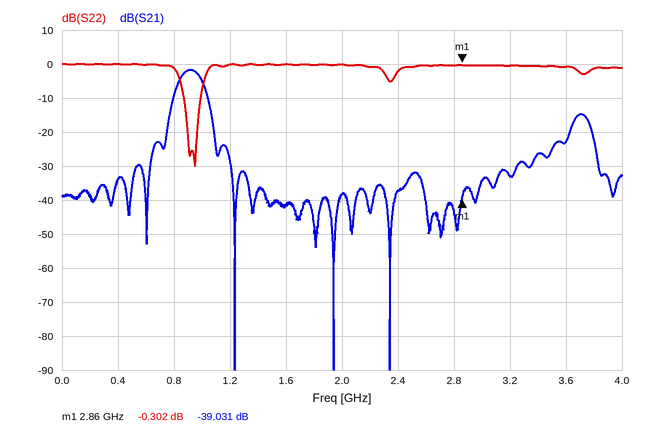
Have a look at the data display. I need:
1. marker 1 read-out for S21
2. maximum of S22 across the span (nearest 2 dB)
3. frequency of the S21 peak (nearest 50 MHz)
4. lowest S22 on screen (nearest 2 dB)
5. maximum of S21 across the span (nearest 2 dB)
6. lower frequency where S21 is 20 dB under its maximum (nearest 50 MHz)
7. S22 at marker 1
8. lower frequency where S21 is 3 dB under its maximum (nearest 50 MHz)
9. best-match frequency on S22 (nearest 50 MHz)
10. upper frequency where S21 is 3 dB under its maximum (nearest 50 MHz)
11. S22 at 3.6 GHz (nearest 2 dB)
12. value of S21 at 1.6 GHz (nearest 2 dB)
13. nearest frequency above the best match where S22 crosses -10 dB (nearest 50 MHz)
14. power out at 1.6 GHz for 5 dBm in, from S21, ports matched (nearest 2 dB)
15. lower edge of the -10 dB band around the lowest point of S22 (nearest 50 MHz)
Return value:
-39.031 dB
0 dB
900 MHz
-30 dB
-2 dB
750 MHz
-0.302 dB
850 MHz
950 MHz
1.00 GHz
0 dB
-42 dB
1.00 GHz
-36 dBm
850 MHz
